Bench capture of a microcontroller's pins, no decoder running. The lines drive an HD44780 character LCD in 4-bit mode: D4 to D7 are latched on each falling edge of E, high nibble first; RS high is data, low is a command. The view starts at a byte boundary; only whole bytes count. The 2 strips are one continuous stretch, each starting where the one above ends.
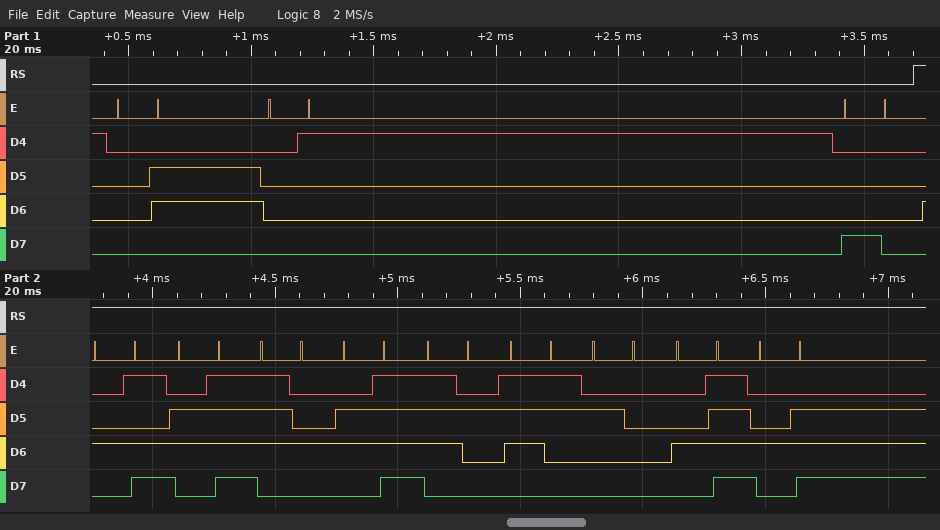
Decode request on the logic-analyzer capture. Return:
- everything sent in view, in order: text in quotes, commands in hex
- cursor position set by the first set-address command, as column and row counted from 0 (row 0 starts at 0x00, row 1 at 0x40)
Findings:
0x06 0x01 0x80 "Motors ON"
column 0, row 0
